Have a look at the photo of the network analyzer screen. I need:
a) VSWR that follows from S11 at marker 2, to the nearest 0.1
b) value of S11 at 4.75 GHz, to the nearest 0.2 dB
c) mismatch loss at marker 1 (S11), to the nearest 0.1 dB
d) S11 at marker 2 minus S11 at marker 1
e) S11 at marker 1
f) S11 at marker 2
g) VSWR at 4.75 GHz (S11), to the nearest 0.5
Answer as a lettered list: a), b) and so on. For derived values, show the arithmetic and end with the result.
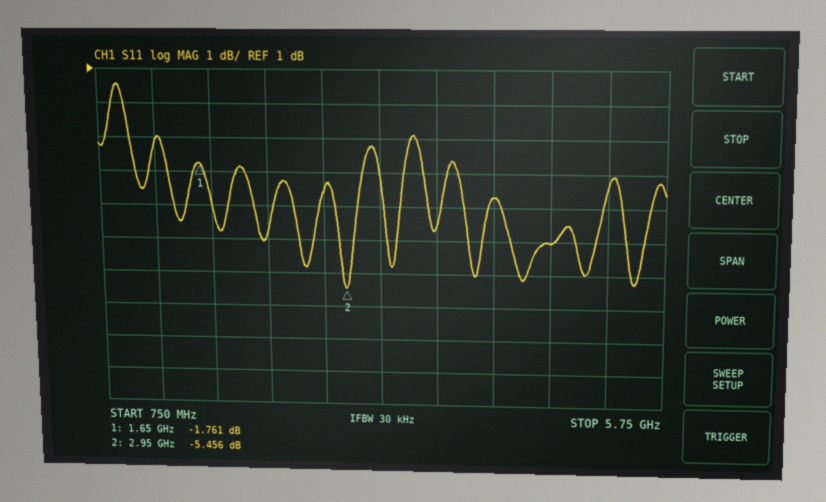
a) (1 + 0.5336)/(1 − 0.5336) ≈ 3.3
b) -4.0 dB
c) −10 log10(1 − 10^(-1.761/10)) ≈ 4.8 dB
d) -5.456 − (-1.761) = -3.695 dB
e) -1.761 dB
f) -5.456 dB
g) |Γ| = 10^(-4/20) = 0.6310; VSWR = (1 + 0.6310)/(1 − 0.6310) ≈ 4.42, so 4.5 to the nearest 0.5
